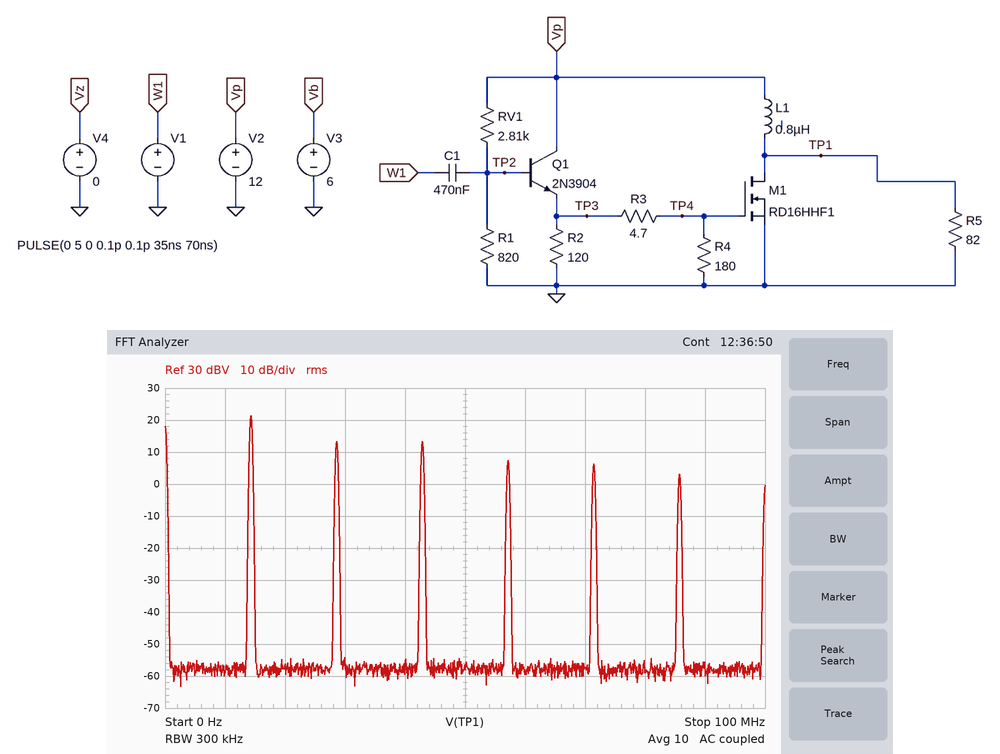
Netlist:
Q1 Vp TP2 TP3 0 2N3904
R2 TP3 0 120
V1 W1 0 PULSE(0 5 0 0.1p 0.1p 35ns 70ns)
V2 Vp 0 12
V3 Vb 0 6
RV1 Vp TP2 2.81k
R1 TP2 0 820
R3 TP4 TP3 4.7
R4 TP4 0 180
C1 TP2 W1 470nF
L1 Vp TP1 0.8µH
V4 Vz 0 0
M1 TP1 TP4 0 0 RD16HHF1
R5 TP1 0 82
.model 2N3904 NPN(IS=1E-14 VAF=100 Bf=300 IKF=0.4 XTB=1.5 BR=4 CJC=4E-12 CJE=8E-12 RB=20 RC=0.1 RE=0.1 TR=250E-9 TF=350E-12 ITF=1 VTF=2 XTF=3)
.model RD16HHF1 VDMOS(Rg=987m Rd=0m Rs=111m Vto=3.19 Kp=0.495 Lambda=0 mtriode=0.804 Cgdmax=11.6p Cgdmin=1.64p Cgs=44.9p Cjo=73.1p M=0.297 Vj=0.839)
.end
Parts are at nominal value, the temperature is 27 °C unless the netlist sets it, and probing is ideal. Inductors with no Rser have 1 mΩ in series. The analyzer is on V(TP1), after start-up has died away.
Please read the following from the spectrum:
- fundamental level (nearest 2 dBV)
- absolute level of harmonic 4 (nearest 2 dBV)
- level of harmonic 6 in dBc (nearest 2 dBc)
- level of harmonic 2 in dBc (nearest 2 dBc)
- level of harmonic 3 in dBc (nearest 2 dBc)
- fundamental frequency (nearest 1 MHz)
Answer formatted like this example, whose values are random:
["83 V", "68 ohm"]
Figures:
["22 dBV", "8 dBV", "-18 dBc", "-8 dBc", "-8 dBc", "14 MHz"]
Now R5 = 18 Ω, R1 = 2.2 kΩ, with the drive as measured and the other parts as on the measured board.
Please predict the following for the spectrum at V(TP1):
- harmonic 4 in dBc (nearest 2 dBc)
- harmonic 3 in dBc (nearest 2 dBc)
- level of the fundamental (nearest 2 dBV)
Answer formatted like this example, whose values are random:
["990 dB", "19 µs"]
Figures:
["-18 dBc", "-10 dBc", "20 dBV"]
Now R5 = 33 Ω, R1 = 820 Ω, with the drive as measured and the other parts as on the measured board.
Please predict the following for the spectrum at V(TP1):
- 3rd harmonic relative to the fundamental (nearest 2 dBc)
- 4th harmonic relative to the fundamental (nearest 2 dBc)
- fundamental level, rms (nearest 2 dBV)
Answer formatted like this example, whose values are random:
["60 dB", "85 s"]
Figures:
["-10 dBc", "-20 dBc", "20 dBV"]
